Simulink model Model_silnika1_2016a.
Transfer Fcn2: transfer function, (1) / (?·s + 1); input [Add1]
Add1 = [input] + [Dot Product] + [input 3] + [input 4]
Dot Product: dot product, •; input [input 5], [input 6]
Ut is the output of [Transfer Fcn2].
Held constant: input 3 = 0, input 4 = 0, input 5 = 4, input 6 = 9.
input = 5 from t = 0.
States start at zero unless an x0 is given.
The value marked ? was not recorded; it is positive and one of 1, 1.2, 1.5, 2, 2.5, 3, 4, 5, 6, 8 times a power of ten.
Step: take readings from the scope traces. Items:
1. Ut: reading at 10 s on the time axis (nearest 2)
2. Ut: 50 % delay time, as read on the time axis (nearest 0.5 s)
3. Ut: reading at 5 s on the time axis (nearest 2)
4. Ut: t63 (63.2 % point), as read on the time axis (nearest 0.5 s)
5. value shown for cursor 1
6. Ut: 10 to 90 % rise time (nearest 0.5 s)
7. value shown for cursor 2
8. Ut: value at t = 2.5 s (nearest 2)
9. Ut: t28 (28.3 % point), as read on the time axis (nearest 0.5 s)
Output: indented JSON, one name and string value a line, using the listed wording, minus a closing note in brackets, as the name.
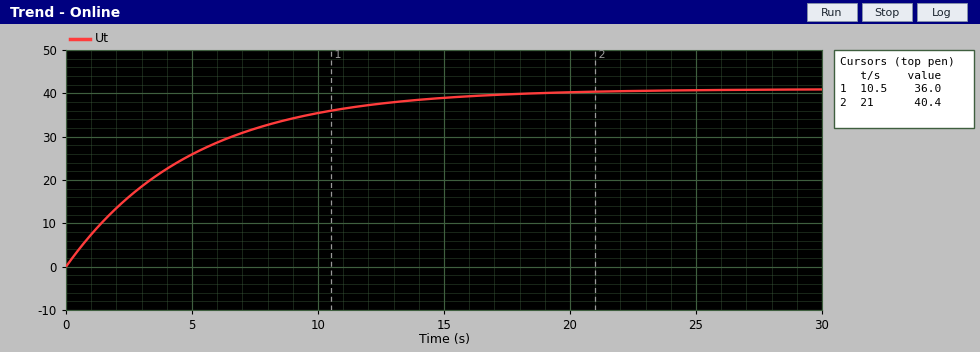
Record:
{
  "Ut: reading at 10 s on the time axis": "36",
  "Ut: 50 % delay time, as read on the time axis": "3.5 s",
  "Ut: reading at 5 s on the time axis": "26",
  "Ut: t63 (63.2 % point), as read on the time axis": "5.0 s",
  "value shown for cursor 1": "36.0",
  "Ut: 10 to 90 % rise time": "11.0 s",
  "value shown for cursor 2": "40.4",
  "Ut: value at t = 2.5 s": "16",
  "Ut: t28 (28.3 % point), as read on the time axis": "1.5 s"
}
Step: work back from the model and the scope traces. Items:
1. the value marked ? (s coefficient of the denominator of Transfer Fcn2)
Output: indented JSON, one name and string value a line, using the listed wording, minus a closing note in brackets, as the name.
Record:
{
  "the value marked ?": "5"
}
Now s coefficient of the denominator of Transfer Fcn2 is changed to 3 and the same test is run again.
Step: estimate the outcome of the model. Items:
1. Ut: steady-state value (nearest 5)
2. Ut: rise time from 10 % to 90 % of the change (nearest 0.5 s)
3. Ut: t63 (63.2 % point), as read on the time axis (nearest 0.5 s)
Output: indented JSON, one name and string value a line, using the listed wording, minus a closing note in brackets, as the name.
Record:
{
  "Ut: steady-state value": "40",
  "Ut: rise time from 10 % to 90 % of the change": "6.5 s",
  "Ut: t63 (63.2 % point), as read on the time axis": "3.0 s"
}
